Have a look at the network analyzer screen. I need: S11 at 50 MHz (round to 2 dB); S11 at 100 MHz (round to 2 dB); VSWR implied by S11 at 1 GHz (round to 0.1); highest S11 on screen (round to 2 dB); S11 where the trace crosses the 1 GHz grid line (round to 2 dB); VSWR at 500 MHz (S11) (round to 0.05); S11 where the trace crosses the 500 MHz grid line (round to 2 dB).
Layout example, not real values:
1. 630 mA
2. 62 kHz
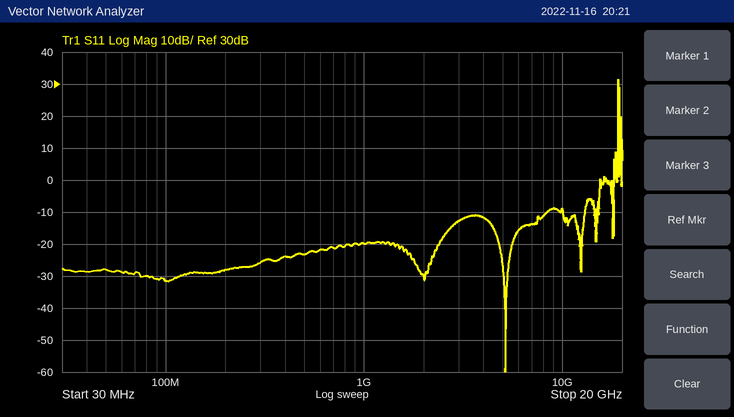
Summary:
1. -28 dB
2. -32 dB
3. 1.2
4. 32 dB
5. -20 dB
6. 1.15
7. -24 dB
